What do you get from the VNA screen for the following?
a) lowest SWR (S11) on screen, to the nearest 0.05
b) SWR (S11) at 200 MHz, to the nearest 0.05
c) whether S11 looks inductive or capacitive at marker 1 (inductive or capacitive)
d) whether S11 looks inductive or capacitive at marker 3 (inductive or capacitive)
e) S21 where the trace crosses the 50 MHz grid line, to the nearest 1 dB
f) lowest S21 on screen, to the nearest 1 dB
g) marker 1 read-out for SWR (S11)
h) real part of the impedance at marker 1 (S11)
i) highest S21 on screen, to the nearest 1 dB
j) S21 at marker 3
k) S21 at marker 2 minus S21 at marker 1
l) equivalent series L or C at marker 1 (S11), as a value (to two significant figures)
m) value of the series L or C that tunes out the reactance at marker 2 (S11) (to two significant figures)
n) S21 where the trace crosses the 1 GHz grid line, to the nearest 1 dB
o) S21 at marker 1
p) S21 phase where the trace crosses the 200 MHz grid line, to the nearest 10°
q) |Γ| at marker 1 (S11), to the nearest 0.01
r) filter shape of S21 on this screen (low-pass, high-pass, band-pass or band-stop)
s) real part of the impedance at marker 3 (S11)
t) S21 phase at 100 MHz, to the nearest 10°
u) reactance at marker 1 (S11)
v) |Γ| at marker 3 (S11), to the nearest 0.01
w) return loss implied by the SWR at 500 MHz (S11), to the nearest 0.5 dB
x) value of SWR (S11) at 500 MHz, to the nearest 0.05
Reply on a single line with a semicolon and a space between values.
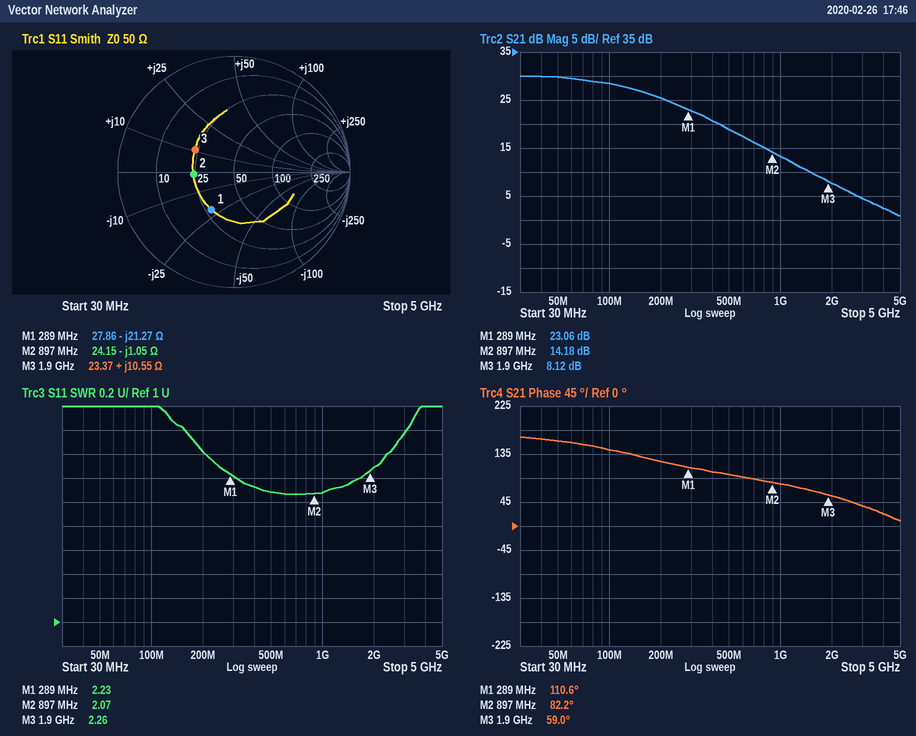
2.05; 2.40; capacitive; inductive; 30 dB; 1 dB; 2.23; 27.86 Ω; 30 dB; 8.12 dB; -8.88 dB; 26 pF; 190 pH; 13 dB; 23.06 dB; 120°; 0.38; low-pass; 23.37 Ω; 140°; -21.27 Ω; 0.39; 9.0 dB; 2.10
